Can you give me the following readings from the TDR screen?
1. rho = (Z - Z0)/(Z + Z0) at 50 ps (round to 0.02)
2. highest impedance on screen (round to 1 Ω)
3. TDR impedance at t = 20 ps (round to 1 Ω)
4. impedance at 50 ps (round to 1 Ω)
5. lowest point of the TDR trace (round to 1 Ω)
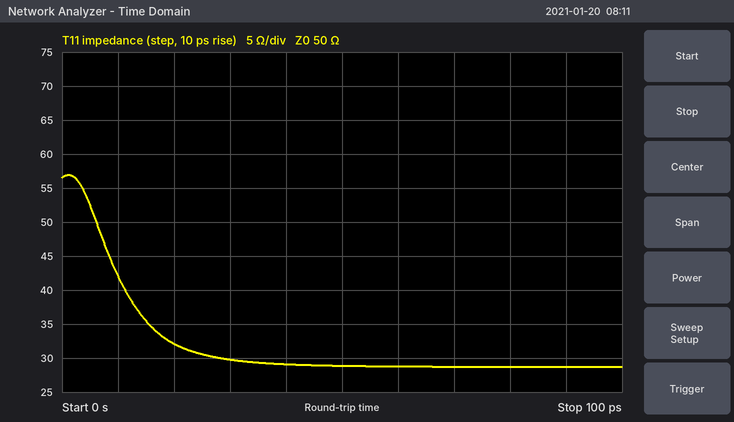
-0.26
57 Ω
32 Ω
29 Ω
29 Ω
